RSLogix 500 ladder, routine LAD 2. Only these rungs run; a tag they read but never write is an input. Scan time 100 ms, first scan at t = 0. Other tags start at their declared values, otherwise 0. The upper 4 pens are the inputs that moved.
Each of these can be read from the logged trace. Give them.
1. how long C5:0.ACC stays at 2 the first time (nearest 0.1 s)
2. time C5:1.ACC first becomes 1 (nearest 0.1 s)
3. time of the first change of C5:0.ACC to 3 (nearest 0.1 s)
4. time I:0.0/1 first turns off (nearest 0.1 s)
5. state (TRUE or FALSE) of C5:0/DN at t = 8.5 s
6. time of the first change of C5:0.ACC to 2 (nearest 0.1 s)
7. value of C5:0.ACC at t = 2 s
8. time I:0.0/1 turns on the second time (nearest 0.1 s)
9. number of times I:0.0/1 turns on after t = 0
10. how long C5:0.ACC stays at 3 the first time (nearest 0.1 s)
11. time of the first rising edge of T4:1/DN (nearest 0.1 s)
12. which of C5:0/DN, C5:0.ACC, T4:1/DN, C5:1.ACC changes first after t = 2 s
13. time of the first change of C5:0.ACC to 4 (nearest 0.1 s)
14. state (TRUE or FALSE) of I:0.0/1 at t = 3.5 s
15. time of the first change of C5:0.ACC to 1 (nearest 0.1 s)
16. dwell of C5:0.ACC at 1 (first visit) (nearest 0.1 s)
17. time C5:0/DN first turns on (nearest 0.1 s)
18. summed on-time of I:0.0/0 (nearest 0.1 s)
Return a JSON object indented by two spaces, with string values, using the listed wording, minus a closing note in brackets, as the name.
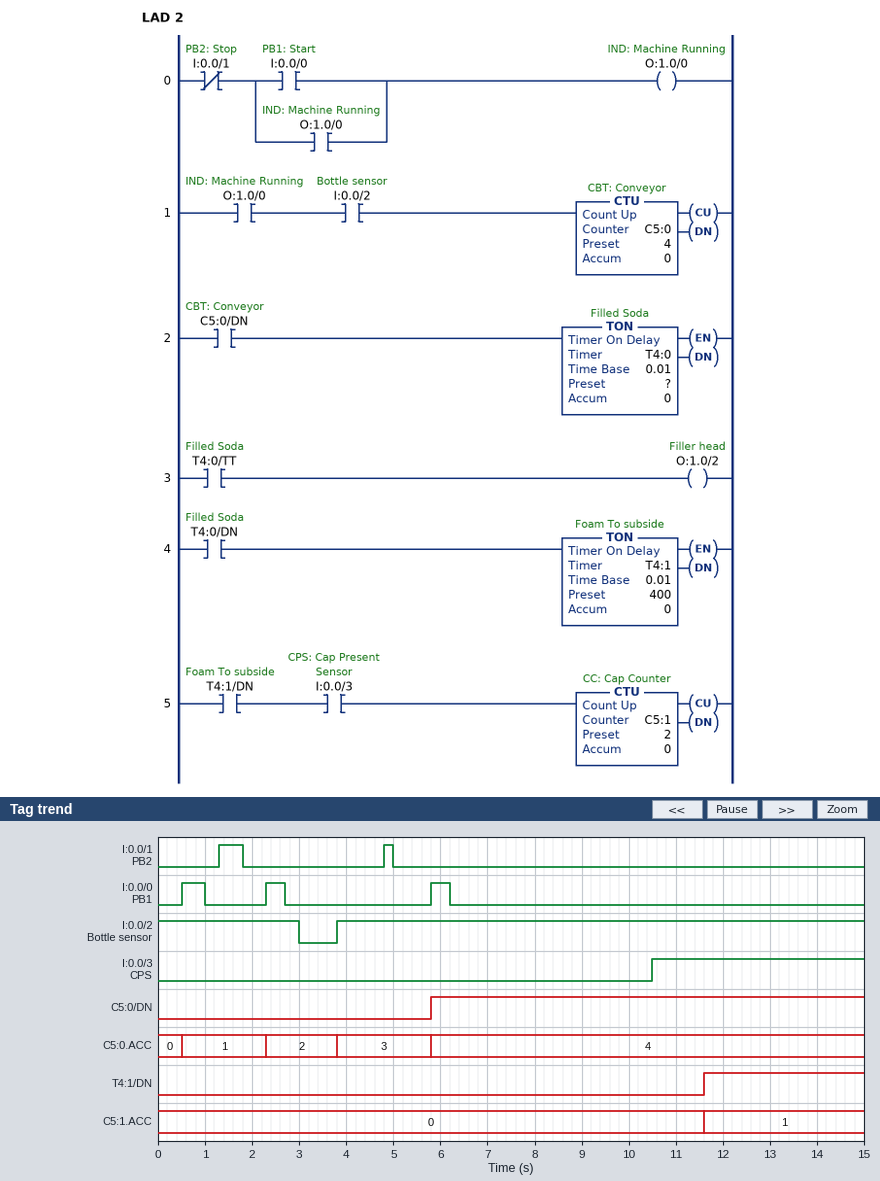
{
  "how long C5:0.ACC stays at 2 the first time": "1.5 s",
  "time C5:1.ACC first becomes 1": "11.6 s",
  "time of the first change of C5:0.ACC to 3": "3.8 s",
  "time I:0.0/1 first turns off": "1.8 s",
  "state (TRUE or FALSE) of C5:0/DN at t = 8.5 s": "TRUE",
  "time of the first change of C5:0.ACC to 2": "2.3 s",
  "value of C5:0.ACC at t = 2 s": "1",
  "time I:0.0/1 turns on the second time": "4.8 s",
  "number of times I:0.0/1 turns on after t = 0": "2",
  "how long C5:0.ACC stays at 3 the first time": "2.0 s",
  "time of the first rising edge of T4:1/DN": "11.6 s",
  "which of C5:0/DN, C5:0.ACC, T4:1/DN, C5:1.ACC changes first after t = 2 s": "C5:0.ACC",
  "time of the first change of C5:0.ACC to 4": "5.8 s",
  "state (TRUE or FALSE) of I:0.0/1 at t = 3.5 s": "FALSE",
  "time of the first change of C5:0.ACC to 1": "0.5 s",
  "dwell of C5:0.ACC at 1 (first visit)": "1.8 s",
  "time C5:0/DN first turns on": "5.8 s",
  "summed on-time of I:0.0/0": "1.3 s"
}
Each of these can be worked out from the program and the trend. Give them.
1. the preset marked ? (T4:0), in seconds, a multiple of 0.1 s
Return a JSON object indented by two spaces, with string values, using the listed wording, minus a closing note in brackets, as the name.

{
  "the preset marked ? (T4:0), in seconds, a multiple of 0.1 s": "1.8 s"
}
